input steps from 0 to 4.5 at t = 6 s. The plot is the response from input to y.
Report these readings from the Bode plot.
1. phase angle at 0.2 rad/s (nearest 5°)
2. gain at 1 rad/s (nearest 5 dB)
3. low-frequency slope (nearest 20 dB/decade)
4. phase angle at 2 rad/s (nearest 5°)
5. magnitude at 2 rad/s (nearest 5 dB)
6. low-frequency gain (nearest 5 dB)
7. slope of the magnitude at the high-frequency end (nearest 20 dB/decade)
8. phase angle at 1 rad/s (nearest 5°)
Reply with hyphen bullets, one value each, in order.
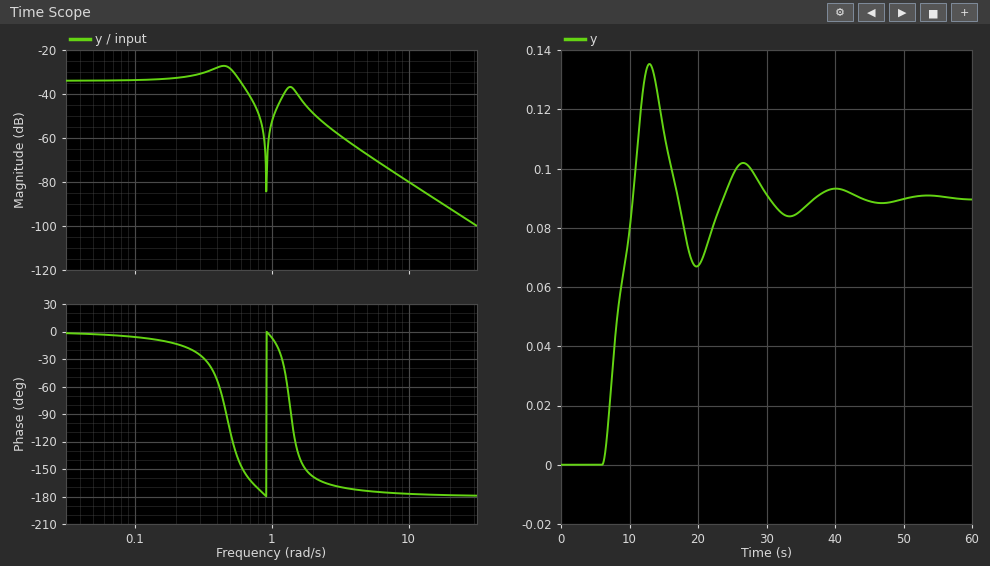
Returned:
- -15°
- -55 dB
- 0 dB/decade
- -160°
- -50 dB
- -35 dB
- -40 dB/decade
- -5°
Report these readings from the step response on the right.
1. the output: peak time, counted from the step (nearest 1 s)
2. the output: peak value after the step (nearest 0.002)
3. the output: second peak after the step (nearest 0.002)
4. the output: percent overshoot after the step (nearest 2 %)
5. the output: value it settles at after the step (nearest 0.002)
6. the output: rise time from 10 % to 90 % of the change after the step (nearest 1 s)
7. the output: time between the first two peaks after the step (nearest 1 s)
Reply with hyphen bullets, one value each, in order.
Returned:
- 7 s
- 0.136
- 0.102
- 50 %
- 0.090
- 3 s
- 14 s
